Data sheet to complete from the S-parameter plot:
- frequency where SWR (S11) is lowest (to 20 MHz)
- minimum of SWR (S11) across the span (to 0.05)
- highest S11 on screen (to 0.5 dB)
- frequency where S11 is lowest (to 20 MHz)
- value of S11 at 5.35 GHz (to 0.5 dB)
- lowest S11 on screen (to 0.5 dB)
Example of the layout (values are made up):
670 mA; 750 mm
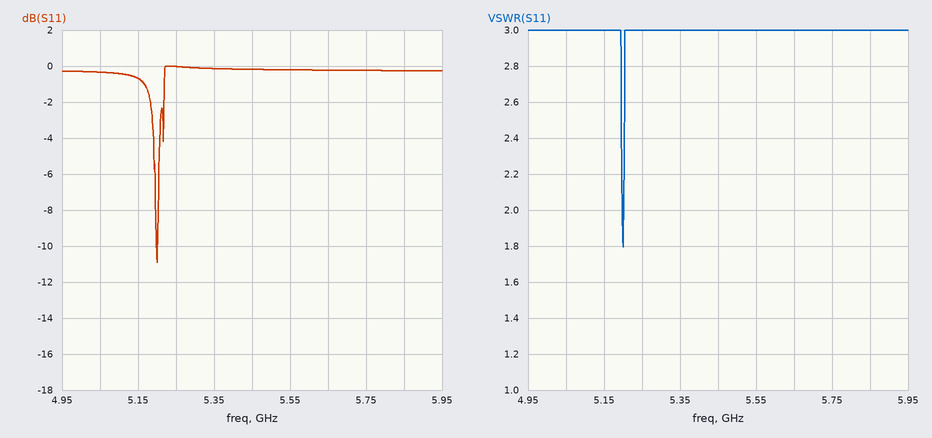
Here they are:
5.20 GHz; 1.80; 0.0 dB; 5.20 GHz; 0.0 dB; -11.0 dB
